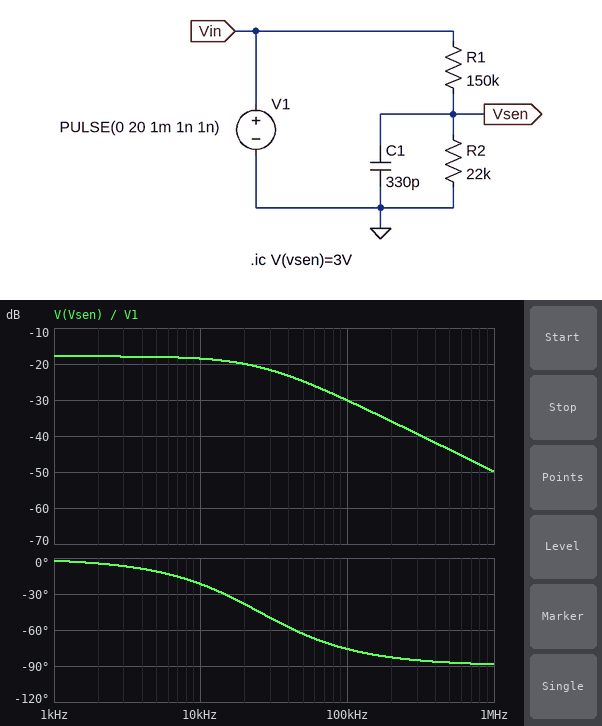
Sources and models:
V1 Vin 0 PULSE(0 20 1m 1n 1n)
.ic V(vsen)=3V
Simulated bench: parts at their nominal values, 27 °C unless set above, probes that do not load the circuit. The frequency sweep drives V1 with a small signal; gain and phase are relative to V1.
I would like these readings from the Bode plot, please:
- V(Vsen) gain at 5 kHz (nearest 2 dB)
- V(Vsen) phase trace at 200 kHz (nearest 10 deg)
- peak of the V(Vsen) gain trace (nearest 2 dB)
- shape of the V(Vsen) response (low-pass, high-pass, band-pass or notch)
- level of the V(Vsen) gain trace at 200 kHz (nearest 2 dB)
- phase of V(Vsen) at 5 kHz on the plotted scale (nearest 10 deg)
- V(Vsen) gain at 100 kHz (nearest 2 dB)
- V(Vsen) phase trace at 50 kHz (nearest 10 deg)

-18 dB
-80 deg
-18 dB
low-pass
-36 dB
-10 deg
-30 dB
-60 deg
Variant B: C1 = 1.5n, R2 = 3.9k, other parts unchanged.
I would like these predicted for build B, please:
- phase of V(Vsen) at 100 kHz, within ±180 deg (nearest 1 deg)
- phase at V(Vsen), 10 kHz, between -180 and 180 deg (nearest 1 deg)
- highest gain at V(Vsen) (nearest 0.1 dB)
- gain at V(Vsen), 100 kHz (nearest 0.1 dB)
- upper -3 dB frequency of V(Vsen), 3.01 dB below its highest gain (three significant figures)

-74 deg
-20 deg
-31.9 dB
-43.3 dB
27.9 kHz
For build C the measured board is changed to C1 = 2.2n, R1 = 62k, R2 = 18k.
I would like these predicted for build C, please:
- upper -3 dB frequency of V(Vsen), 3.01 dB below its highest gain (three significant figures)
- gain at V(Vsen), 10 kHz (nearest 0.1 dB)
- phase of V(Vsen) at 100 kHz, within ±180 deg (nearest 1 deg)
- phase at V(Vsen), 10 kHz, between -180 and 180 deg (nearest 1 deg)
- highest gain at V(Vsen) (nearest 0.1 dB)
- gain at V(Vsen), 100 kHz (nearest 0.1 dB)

5.19 kHz
-19.7 dB
-87 deg
-63 deg
-13.0 dB
-38.7 dB
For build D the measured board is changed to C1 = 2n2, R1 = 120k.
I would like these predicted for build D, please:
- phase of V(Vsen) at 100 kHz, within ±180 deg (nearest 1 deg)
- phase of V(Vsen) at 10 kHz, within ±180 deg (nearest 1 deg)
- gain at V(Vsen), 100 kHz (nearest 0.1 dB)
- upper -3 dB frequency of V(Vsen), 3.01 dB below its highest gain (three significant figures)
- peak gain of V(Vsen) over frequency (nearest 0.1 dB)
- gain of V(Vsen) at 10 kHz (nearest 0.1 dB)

-88 deg
-69 deg
-44.4 dB
3.89 kHz
-16.2 dB
-25.0 dB
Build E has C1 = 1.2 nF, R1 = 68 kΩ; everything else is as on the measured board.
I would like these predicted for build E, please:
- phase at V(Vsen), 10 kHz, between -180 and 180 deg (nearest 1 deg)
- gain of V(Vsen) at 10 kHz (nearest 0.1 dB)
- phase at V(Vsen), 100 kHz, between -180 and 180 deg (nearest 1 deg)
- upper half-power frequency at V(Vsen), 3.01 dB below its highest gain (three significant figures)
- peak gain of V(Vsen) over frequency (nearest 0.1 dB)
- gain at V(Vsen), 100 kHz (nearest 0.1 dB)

-51 deg
-16.3 dB
-85 deg
7.98 kHz
-12.2 dB
-34.2 dB
